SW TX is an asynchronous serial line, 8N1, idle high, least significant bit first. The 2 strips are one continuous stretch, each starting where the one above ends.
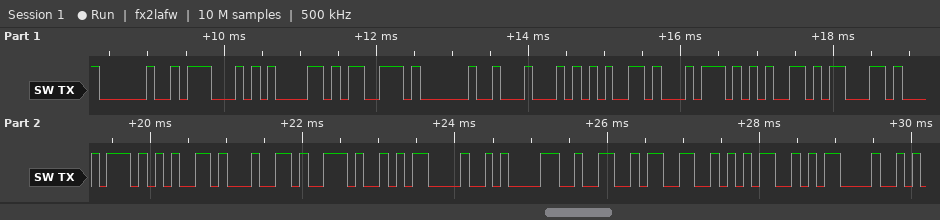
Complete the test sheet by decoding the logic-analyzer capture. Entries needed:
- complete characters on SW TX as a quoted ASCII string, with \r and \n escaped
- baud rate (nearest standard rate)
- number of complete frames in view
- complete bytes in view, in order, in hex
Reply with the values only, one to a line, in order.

" Gas Detected.\r\n235\r"
9600 baud
20
20 47 61 73 20 44 65 74 65 63 74 65 64 2E 0D 0A 32 33 35 0D
